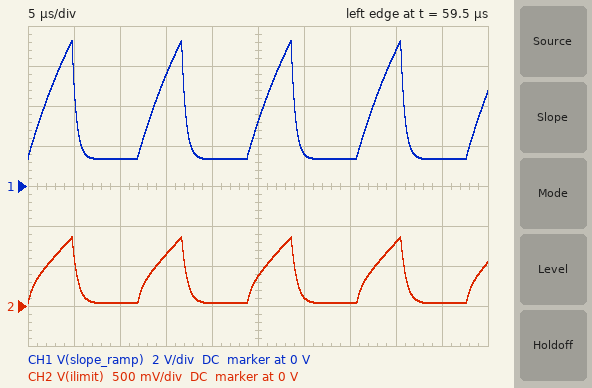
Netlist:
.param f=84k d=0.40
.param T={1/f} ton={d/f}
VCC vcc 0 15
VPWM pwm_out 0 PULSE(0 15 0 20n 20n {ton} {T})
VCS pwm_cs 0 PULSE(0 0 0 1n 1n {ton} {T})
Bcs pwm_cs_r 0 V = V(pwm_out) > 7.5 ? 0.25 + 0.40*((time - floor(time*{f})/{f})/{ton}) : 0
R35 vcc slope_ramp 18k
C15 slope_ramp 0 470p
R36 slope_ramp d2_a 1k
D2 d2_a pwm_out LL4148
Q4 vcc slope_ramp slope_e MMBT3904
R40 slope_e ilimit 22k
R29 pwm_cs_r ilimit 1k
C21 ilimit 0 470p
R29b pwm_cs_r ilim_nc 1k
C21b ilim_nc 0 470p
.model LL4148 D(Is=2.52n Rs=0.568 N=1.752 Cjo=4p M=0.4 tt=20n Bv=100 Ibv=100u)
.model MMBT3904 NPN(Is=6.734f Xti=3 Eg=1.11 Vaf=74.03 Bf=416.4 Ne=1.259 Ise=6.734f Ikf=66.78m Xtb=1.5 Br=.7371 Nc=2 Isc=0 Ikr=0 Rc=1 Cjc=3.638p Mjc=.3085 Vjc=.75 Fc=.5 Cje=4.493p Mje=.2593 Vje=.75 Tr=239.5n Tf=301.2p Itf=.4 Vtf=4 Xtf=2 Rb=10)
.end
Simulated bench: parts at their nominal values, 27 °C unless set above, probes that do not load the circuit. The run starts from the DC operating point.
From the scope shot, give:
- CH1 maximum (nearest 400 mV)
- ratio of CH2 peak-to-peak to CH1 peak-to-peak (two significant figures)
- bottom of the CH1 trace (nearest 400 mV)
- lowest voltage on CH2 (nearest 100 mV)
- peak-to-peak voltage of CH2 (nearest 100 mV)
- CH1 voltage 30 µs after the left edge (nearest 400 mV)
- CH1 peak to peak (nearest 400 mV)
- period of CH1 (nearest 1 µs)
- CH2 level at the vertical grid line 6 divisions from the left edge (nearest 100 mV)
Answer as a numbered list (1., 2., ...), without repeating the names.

1. 7.2 V
2. 0.14
3. 1.2 V
4. 0 V
5. 800 mV
6. 1.6 V
7. 6.0 V
8. 12 µs
9. 100 mV
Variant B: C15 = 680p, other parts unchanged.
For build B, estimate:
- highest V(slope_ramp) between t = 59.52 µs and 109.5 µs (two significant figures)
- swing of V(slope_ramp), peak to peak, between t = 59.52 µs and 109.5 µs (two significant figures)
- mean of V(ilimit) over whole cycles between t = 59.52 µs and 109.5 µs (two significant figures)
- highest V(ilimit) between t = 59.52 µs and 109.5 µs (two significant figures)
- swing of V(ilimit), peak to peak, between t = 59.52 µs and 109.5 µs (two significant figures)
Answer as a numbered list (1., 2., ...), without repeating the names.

1. 5.8 V
2. 4.4 V
3. 260 mV
4. 800 mV
5. 760 mV
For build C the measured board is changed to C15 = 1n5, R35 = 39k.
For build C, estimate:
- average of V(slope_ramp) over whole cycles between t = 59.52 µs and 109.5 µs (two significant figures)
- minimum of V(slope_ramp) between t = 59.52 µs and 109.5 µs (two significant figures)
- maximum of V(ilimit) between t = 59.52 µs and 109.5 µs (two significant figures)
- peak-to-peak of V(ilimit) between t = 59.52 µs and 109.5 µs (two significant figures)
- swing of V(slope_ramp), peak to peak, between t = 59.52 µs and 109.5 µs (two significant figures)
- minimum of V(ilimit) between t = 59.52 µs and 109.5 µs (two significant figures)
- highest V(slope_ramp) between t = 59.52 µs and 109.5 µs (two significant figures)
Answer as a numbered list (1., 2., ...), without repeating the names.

1. 1.3 V
2. 910 mV
3. 650 mV
4. 630 mV
5. 1.1 V
6. 16 mV
7. 2.0 V
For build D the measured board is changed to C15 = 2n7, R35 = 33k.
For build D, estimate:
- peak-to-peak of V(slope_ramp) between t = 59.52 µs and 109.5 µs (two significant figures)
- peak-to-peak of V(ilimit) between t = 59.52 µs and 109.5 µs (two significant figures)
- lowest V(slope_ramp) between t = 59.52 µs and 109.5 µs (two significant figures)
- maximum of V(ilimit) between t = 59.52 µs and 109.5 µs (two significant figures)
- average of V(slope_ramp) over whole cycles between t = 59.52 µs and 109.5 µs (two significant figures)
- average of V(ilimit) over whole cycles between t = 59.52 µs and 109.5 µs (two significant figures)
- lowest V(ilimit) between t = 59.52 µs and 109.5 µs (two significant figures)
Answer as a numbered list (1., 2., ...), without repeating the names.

1. 740 mV
2. 620 mV
3. 1.0 V
4. 640 mV
5. 1.3 V
6. 210 mV
7. 21 mV
